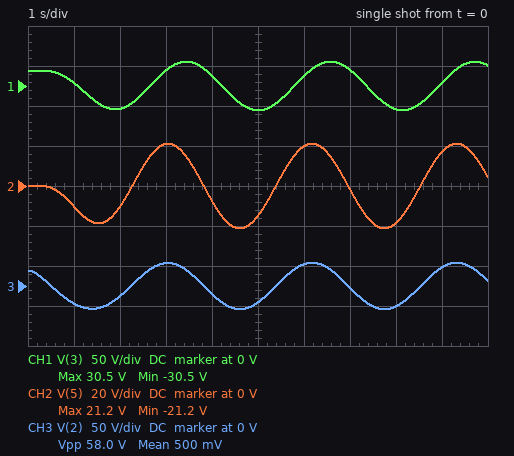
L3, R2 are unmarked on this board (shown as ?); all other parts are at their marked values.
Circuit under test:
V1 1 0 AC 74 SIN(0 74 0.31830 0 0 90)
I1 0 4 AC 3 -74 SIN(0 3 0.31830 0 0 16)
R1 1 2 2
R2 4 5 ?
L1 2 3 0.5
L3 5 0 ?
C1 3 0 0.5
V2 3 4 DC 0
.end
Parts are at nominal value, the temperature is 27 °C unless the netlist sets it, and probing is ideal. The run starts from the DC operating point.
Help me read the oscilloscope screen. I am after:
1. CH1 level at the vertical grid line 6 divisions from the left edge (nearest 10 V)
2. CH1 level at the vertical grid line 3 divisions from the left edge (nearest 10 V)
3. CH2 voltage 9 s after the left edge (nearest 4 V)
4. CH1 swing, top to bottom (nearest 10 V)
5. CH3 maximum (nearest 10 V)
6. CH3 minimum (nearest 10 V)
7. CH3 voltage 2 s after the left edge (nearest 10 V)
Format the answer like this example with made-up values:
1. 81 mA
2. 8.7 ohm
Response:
1. 10 V
2. 20 V
3. 16 V
4. 60 V
5. 30 V
6. -30 V
7. -10 V
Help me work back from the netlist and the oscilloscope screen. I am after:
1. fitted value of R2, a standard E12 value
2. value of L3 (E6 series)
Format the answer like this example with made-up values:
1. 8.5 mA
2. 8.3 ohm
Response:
1. 0.68 Ω
2. 330 mH
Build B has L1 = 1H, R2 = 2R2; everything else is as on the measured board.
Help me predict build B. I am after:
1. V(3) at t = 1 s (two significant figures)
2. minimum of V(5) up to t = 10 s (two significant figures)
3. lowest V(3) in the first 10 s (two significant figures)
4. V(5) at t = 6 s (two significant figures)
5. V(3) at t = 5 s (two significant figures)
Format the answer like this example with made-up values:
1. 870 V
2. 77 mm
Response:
1. 29 V
2. -9.1 V
3. -33 V
4. 5.8 V
5. -17 V
